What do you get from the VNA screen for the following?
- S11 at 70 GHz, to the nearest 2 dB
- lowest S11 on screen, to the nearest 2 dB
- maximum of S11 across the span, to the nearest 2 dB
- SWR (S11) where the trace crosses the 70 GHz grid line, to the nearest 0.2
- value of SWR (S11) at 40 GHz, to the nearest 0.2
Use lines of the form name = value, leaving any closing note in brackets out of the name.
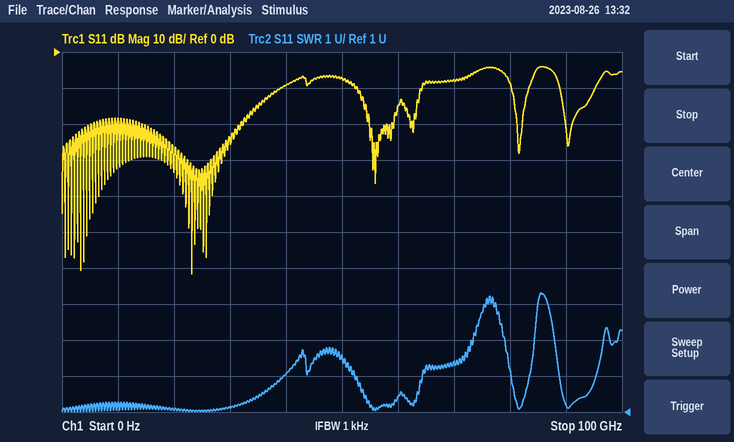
S11 at 70 GHz, to the nearest 2 dB = -8 dB
lowest S11 on screen, to the nearest 2 dB = -62 dB
maximum of S11 across the span, to the nearest 2 dB = -4 dB
SWR (S11) where the trace crosses the 70 GHz grid line, to the nearest 0.2 = 2.4
value of SWR (S11) at 40 GHz, to the nearest 0.2 = 2.0
